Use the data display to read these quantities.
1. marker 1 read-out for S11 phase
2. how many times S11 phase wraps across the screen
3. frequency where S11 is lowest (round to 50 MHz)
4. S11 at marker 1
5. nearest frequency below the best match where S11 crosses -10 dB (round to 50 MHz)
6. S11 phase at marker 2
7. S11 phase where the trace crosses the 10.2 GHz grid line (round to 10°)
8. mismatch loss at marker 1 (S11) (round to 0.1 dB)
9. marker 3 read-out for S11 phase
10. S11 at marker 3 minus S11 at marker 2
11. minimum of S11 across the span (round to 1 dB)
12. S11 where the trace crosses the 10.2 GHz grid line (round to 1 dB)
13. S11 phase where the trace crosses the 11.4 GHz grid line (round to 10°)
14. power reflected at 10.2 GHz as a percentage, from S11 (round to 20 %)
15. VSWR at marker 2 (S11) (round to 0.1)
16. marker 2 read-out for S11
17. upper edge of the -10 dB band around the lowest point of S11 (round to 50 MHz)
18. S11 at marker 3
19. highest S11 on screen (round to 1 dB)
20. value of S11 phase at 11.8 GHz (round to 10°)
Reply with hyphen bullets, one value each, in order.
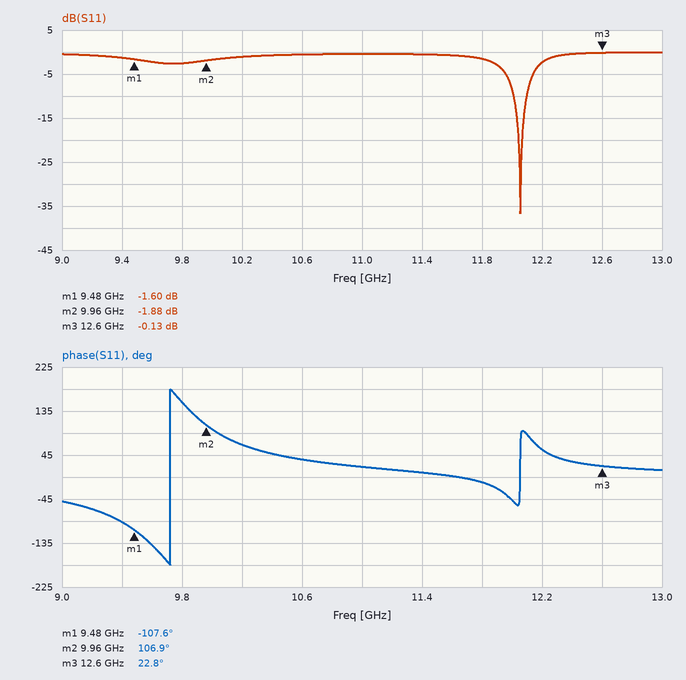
- -107.6°
- 1
- 12.05 GHz
- -1.60 dB
- 12.00 GHz
- 106.9°
- 70°
- 5.1 dB
- 22.8°
- 1.75 dB
- -37 dB
- -1 dB
- 10°
- 80 %
- 9.3
- -1.88 dB
- 12.10 GHz
- -0.13 dB
- 0 dB
- -10°
